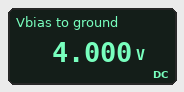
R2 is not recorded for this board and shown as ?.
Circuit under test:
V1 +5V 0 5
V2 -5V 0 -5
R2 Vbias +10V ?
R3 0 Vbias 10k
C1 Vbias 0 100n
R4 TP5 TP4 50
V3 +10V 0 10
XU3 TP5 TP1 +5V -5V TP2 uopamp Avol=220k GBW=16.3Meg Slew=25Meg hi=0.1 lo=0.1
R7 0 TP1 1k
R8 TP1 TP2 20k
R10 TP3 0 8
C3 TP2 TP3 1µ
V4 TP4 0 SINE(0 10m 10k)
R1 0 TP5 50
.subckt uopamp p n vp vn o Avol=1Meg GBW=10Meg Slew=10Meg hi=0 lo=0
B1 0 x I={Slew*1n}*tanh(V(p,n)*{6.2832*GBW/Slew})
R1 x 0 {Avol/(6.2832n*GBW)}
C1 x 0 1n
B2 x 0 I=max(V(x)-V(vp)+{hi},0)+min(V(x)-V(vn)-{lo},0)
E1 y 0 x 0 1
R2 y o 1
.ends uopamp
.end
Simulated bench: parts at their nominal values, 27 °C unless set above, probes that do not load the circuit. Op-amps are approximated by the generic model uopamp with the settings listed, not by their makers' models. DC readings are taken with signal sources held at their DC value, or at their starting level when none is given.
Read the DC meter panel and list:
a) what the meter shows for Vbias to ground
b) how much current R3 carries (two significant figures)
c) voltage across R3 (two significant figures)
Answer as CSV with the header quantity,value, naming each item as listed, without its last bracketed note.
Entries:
quantity,value
what the meter shows for Vbias to ground,4.000 V
how much current R3 carries,400 µA
voltage across R3,4.0 V
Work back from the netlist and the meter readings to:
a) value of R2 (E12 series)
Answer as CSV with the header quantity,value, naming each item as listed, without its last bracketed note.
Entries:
quantity,value
value of R2,15 kΩ
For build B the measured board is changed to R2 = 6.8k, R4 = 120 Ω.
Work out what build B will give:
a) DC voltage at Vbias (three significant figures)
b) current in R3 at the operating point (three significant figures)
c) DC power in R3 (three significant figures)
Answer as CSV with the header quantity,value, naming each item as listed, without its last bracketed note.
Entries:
quantity,value
DC voltage at Vbias,5.95 V
current in R3 at the operating point,595 µA
DC power in R3,3.54 mW
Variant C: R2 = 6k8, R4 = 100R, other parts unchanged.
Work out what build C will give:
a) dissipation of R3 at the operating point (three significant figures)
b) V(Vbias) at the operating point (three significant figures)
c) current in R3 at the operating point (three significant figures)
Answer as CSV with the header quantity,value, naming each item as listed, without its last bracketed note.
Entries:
quantity,value
dissipation of R3 at the operating point,3.54 mW
V(Vbias) at the operating point,5.95 V
current in R3 at the operating point,595 µA
